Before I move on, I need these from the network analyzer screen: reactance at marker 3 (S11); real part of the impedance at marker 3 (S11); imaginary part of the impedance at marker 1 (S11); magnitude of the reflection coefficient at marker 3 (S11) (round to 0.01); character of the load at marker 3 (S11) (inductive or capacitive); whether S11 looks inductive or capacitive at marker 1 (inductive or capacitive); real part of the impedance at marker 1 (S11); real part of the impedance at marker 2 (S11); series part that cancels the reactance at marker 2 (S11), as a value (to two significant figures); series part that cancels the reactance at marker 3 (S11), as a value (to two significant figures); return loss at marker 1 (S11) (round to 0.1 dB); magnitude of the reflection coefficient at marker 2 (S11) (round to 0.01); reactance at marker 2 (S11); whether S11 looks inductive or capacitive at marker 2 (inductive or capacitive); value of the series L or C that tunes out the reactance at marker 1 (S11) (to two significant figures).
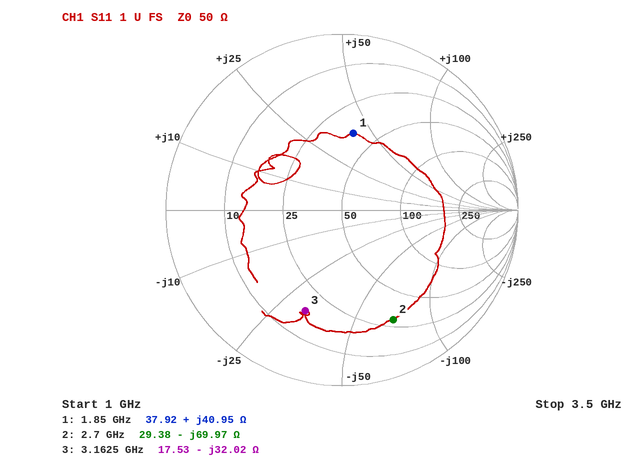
-32.02 Ω
17.53 Ω
+40.95 Ω
0.61
capacitive
inductive
37.92 Ω
29.38 Ω
4.1 nH
1.6 nH
7.1 dB
0.69
-69.97 Ω
capacitive
2.1 pF
